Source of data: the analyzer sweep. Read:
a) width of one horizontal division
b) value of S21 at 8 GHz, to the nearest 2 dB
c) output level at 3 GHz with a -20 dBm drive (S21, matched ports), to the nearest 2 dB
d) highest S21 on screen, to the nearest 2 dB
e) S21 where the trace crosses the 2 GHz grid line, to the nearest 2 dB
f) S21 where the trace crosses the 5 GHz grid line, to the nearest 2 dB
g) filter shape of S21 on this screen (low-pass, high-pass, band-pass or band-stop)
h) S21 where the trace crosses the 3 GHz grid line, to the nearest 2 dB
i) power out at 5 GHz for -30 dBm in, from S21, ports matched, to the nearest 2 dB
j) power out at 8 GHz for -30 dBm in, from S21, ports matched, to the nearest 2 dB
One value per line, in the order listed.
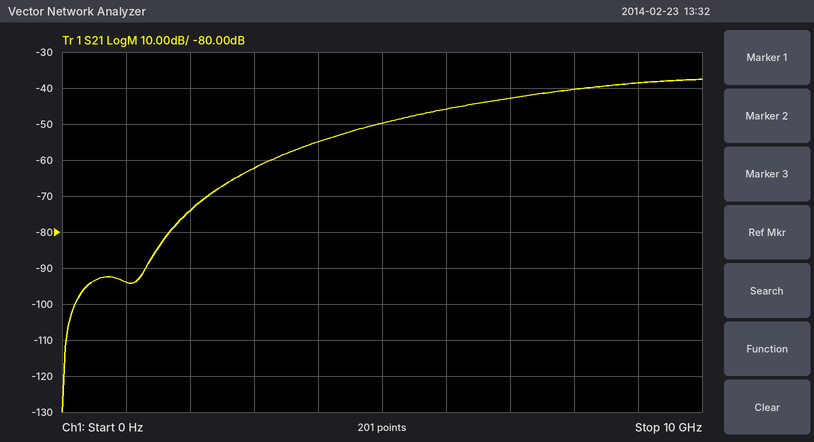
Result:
1 GHz
-40 dB
-82 dBm
-38 dB
-74 dB
-50 dB
high-pass
-62 dB
-80 dBm
-70 dBm
